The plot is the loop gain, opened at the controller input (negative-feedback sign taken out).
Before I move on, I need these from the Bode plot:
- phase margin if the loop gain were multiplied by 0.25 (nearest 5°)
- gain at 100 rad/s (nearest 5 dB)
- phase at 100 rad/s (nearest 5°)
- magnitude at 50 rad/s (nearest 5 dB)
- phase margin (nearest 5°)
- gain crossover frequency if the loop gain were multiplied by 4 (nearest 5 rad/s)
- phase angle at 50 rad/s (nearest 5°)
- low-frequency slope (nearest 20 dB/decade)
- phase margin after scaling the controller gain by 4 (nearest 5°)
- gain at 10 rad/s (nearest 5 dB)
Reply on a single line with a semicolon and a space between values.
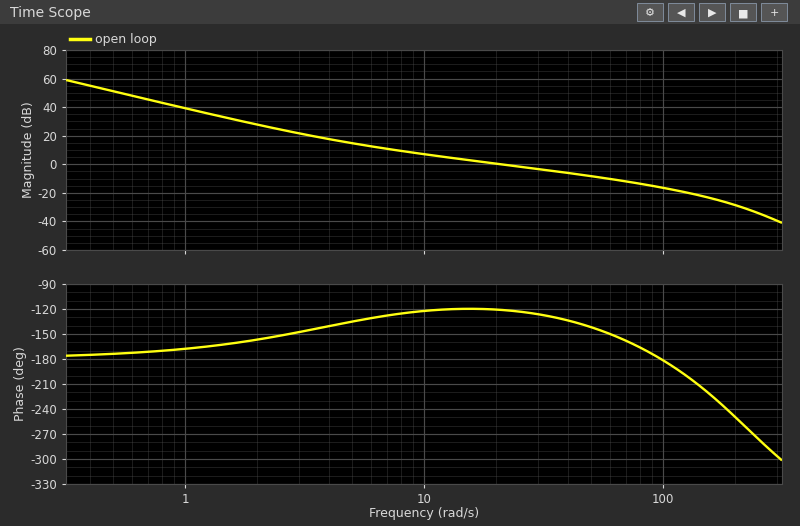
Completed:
50°; -15 dB; -180°; -10 dB; 60°; 70 rad/s; -140°; -40 dB/decade; 20°; 5 dB
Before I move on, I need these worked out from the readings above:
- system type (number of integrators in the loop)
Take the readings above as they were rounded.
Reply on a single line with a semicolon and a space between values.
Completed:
2
